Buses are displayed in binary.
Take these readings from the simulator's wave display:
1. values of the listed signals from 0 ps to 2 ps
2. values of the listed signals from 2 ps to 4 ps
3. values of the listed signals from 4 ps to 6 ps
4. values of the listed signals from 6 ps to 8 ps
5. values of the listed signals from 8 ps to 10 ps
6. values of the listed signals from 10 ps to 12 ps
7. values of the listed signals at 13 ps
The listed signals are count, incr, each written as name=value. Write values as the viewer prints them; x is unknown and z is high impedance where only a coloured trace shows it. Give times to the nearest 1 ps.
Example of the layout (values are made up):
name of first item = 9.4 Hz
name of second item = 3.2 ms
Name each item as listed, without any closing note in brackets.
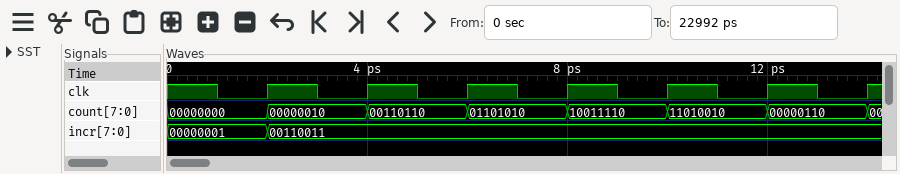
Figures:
values of the listed signals from 0 ps to 2 ps = count=00000000, incr=00000001
values of the listed signals from 2 ps to 4 ps = count=00000010, incr=00110011
values of the listed signals from 4 ps to 6 ps = count=00110110, incr=00110011
values of the listed signals from 6 ps to 8 ps = count=01101010, incr=00110011
values of the listed signals from 8 ps to 10 ps = count=10011110, incr=00110011
values of the listed signals from 10 ps to 12 ps = count=11010010, incr=00110011
values of the listed signals at 13 ps = count=00000110, incr=00110011
